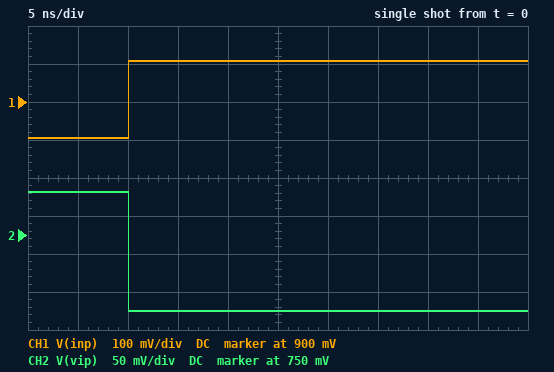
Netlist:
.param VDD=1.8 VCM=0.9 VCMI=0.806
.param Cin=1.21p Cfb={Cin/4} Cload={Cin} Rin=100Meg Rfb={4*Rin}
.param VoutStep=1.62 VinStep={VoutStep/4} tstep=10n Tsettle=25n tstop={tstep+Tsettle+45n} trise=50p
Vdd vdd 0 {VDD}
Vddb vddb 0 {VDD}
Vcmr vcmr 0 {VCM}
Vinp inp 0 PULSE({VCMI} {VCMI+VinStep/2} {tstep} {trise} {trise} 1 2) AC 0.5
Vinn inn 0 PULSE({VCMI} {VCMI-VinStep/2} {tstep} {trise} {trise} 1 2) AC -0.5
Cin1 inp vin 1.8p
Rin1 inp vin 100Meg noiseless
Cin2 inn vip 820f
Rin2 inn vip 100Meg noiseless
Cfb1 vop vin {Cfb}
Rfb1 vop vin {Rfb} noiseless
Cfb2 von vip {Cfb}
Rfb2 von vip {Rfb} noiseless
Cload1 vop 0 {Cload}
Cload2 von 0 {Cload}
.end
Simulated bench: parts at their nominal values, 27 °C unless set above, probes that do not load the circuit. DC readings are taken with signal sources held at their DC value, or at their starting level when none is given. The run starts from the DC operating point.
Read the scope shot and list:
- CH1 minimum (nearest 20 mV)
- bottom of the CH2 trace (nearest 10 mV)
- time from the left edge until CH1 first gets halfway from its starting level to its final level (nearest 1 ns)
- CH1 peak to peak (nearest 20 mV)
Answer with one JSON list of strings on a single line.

["800 mV", "650 mV", "10 ns", "200 mV"]
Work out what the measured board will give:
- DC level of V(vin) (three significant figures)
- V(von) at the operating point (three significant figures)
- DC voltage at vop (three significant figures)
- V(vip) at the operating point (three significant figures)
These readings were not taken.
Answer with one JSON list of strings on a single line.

["806 mV", "806 mV", "806 mV", "806 mV"]
